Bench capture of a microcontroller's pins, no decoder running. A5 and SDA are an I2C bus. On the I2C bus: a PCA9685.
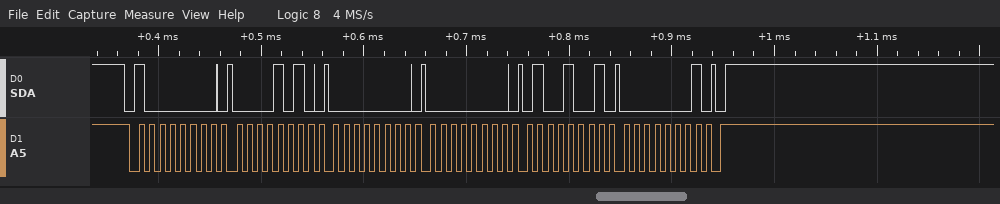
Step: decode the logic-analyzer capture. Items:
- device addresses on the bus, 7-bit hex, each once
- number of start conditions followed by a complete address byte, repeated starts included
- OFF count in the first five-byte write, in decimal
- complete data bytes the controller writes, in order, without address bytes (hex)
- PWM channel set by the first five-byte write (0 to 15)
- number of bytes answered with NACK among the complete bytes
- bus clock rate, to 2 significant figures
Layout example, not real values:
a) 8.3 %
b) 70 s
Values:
a) 0x40
b) 1
c) 329
d) 0A 00 00 49 01
e) 1
f) 0
g) 100 kHz
